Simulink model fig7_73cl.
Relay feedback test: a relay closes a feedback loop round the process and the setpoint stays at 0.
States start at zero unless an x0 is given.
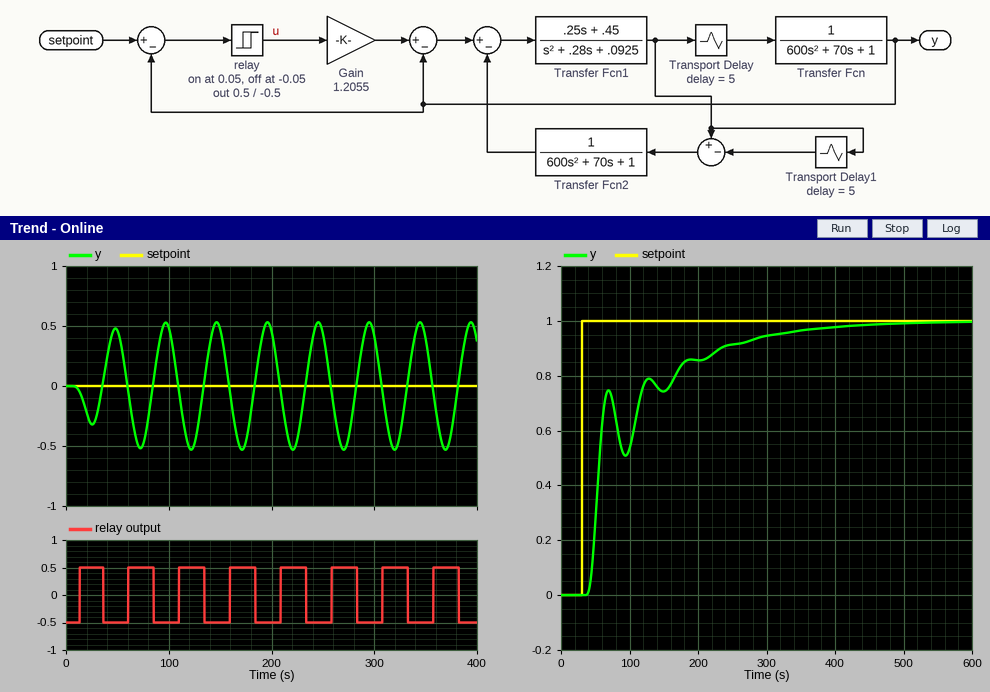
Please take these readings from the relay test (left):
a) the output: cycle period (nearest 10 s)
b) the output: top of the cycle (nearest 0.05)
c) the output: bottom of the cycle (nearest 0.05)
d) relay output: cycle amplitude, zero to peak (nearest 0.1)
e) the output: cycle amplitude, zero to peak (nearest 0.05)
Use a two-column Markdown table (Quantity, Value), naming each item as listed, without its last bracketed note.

| Quantity | Value |
|---|---|
| the output: cycle period | 50 s |
| the output: top of the cycle | 0.55 |
| the output: bottom of the cycle | -0.55 |
| relay output: cycle amplitude, zero to peak | 0.5 |
| the output: cycle amplitude, zero to peak | 0.55 |
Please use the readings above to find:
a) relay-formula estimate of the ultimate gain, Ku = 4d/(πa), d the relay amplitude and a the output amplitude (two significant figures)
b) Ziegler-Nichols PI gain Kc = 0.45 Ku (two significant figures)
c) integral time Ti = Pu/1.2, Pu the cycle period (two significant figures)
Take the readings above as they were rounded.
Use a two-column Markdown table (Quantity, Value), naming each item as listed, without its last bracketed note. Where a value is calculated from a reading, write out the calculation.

| Quantity | Value |
|---|---|
| relay-formula estimate of the ultimate gain, Ku = 4d/(πa), d the relay amplitude and a the output amplitude | 4 × 0.5 / (π × 0.55) = 1.2 |
| Ziegler-Nichols PI gain Kc = 0.45 Ku | 0.45 × 1.2 = 0.54 |
| integral time Ti = Pu/1.2, Pu the cycle period | 50 / 1.2 = 42 s |
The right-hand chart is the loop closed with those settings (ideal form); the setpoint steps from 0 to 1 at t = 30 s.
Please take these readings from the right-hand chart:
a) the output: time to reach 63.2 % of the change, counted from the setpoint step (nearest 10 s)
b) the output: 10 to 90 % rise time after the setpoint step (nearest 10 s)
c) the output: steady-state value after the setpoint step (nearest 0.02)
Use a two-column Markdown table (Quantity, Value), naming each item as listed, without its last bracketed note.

| Quantity | Value |
|---|---|
| the output: time to reach 63.2 % of the change, counted from the setpoint step | 30 s |
| the output: 10 to 90 % rise time after the setpoint step | 190 s |
| the output: steady-state value after the setpoint step | 1.00 |
